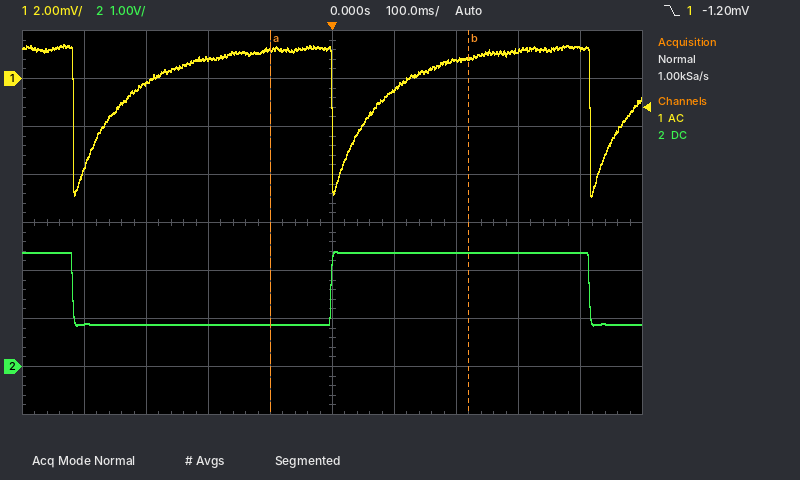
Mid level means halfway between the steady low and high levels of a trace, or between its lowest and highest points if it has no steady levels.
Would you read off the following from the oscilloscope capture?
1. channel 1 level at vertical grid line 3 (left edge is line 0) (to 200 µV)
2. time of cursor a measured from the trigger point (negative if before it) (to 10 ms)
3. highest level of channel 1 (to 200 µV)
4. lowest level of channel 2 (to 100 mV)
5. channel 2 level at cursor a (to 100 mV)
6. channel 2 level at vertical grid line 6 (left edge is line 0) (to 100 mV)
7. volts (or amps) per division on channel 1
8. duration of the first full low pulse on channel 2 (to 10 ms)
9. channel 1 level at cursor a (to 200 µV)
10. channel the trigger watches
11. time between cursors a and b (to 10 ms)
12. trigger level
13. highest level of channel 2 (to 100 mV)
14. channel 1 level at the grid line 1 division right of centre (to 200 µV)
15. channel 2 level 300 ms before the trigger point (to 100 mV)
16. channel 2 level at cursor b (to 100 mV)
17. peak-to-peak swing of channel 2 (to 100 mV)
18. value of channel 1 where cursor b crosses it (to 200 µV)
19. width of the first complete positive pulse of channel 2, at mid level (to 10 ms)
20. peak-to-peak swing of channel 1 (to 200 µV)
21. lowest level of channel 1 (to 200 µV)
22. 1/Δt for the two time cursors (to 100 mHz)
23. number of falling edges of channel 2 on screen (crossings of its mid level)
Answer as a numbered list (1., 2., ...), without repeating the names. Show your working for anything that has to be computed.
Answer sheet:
1. 800 µV
2. -100 ms
3. 1.4 mV
4. 900 mV
5. 900 mV
6. 2.4 V
7. 2 mV
8. 420 ms
9. 1.2 mV
10. channel 1
11. 320 ms
12. -1.20 mV
13. 2.4 V
14. -400 µV
15. 900 mV
16. 2.4 V
17. 2.4 V − (900 mV) = 1.5 V
18. 800 µV
19. 420 ms
20. 1.4 mV − (-5.0 mV) = 6.4 mV
21. -5.0 mV
22. 1 / 320 ms ≈ 3.1 Hz
23. 2
